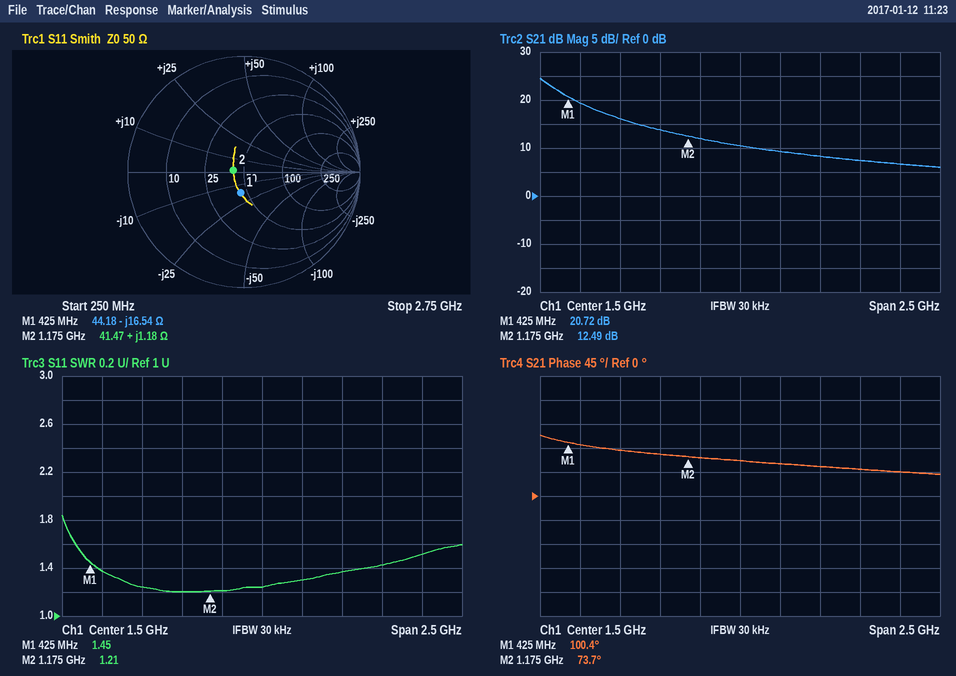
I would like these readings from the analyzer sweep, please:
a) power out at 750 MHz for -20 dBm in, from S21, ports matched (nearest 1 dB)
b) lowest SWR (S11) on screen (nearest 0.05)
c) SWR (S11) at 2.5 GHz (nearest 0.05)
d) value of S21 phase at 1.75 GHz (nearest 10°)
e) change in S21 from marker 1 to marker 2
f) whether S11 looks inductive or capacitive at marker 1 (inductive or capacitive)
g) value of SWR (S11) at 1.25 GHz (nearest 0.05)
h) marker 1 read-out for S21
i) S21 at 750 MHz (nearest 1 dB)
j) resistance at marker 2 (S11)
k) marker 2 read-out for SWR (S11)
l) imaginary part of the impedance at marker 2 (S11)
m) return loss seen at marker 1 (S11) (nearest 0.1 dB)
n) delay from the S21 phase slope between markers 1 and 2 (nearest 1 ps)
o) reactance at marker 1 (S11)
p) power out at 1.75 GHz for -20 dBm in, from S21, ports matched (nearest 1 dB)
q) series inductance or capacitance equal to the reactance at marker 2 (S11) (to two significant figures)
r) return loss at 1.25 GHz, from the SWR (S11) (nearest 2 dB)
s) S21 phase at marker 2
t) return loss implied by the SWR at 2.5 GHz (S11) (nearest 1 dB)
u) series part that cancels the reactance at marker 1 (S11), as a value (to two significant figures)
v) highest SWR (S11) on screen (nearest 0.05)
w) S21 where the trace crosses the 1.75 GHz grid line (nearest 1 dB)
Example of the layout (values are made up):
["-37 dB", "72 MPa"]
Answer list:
["-4 dBm", "1.20", "1.50", "60°", "-8.23 dB", "capacitive", "1.20", "20.72 dB", "16 dB", "41.47 Ω", "1.21", "+1.18 Ω", "14.7 dB", "99 ps", "-16.54 Ω", "-11 dBm", "160 pH", "20 dB", "73.7°", "14 dB", "6.2 nH", "1.85", "9 dB"]
